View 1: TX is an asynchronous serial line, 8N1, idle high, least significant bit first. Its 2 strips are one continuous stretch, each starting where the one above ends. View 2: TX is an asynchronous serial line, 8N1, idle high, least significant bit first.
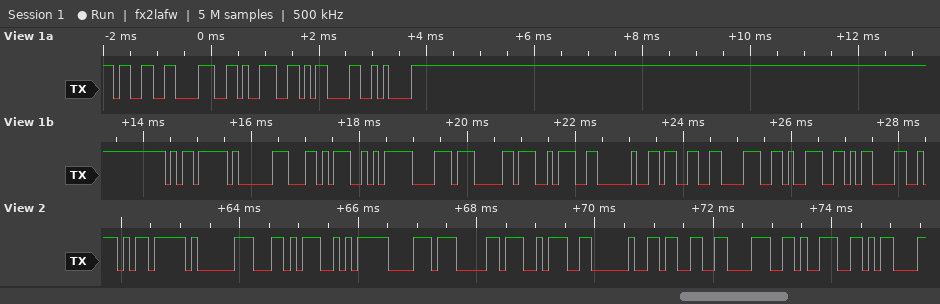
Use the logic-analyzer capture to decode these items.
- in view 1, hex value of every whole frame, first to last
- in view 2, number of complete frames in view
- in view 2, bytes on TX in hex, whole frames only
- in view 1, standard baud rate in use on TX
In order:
33 38 39 0D 0A ED 81 AC EA B8 B0 3A 20 33 38 39 0D
12
ED 81 AC EA B8 B0 3A 20 33 38 39 0D
9600 baud
